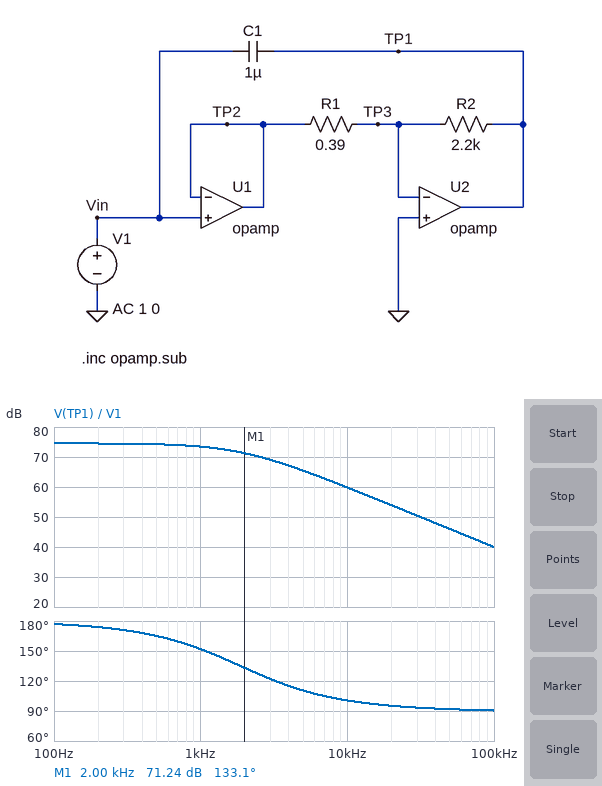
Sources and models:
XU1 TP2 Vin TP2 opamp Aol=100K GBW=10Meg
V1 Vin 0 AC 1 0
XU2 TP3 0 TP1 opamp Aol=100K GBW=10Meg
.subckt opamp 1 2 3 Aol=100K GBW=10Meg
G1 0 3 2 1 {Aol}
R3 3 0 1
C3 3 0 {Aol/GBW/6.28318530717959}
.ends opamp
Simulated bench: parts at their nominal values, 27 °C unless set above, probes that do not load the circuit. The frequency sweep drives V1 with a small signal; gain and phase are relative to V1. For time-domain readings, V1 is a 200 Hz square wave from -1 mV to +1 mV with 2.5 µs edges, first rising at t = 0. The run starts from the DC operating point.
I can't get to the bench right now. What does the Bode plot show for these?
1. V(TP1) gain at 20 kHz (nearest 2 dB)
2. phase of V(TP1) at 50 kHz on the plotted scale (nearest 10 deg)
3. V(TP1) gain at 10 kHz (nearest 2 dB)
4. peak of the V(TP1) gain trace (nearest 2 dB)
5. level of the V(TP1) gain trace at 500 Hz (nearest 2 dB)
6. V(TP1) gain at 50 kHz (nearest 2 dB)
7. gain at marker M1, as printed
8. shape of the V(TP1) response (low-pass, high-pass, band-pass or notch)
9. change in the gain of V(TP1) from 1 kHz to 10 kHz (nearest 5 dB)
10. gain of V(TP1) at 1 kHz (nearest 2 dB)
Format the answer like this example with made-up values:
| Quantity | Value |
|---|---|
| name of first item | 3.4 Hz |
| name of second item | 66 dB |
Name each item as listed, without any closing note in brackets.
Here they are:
| Quantity | Value |
|---|---|
| V(TP1) gain at 20 kHz | 54 dB |
| phase of V(TP1) at 50 kHz on the plotted scale | 90 deg |
| V(TP1) gain at 10 kHz | 60 dB |
| peak of the V(TP1) gain trace | 74 dB |
| level of the V(TP1) gain trace at 500 Hz | 74 dB |
| V(TP1) gain at 50 kHz | 46 dB |
| gain at marker M1, as printed | 71.24 dB |
| shape of the V(TP1) response | low-pass |
| change in the gain of V(TP1) from 1 kHz to 10 kHz | -15 dB |
| gain of V(TP1) at 1 kHz | 74 dB |
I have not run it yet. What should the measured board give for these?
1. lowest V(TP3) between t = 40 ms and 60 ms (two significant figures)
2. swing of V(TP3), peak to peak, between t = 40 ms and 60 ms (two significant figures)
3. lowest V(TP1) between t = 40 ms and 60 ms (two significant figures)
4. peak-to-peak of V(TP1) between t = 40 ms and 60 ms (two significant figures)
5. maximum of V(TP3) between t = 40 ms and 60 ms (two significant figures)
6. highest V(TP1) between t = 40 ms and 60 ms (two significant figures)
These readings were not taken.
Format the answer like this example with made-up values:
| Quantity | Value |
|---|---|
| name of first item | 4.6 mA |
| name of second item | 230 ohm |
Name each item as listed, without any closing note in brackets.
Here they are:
| Quantity | Value |
|---|---|
| lowest V(TP3) between t = 40 ms and 60 ms | -1.9 mV |
| swing of V(TP3), peak to peak, between t = 40 ms and 60 ms | 3.8 mV |
| lowest V(TP1) between t = 40 ms and 60 ms | -5.3 V |
| peak-to-peak of V(TP1) between t = 40 ms and 60 ms | 11 V |
| maximum of V(TP3) between t = 40 ms and 60 ms | 1.9 mV |
| highest V(TP1) between t = 40 ms and 60 ms | 5.3 V |
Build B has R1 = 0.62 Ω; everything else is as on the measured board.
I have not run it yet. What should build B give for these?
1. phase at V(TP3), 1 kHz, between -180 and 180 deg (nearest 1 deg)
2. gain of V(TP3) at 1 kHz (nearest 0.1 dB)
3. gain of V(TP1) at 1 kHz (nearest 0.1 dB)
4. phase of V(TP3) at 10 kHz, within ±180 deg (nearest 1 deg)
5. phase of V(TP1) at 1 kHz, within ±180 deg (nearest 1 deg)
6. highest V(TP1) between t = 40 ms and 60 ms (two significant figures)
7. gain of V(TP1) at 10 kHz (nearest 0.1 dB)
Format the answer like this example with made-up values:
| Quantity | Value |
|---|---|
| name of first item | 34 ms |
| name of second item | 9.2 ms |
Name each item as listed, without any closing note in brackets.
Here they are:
| Quantity | Value |
|---|---|
| phase at V(TP3), 1 kHz, between -180 and 180 deg | 65 deg |
| gain of V(TP3) at 1 kHz | -9.7 dB |
| gain of V(TP1) at 1 kHz | 70.2 dB |
| phase of V(TP3) at 10 kHz, within ±180 deg | 16 deg |
| phase of V(TP1) at 1 kHz, within ±180 deg | 161 deg |
| highest V(TP1) between t = 40 ms and 60 ms | 3.4 V |
| gain of V(TP1) at 10 kHz | 59.6 dB |
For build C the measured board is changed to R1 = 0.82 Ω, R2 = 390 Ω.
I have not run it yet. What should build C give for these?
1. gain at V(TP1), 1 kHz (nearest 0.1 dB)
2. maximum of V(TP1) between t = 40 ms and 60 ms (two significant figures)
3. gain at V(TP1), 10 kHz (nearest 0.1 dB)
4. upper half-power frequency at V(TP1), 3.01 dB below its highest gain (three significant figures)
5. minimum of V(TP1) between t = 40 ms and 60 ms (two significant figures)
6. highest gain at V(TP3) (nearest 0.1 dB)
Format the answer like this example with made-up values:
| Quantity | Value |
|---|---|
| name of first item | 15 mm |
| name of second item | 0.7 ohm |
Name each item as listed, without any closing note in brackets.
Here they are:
| Quantity | Value |
|---|---|
| gain at V(TP1), 1 kHz | 53.5 dB |
| maximum of V(TP1) between t = 40 ms and 60 ms | 470 mV |
| gain at V(TP1), 10 kHz | 52.6 dB |
| upper half-power frequency at V(TP1), 3.01 dB below its highest gain | 21.1 kHz |
| minimum of V(TP1) between t = 40 ms and 60 ms | -470 mV |
| highest gain at V(TP3) | 0 dB |
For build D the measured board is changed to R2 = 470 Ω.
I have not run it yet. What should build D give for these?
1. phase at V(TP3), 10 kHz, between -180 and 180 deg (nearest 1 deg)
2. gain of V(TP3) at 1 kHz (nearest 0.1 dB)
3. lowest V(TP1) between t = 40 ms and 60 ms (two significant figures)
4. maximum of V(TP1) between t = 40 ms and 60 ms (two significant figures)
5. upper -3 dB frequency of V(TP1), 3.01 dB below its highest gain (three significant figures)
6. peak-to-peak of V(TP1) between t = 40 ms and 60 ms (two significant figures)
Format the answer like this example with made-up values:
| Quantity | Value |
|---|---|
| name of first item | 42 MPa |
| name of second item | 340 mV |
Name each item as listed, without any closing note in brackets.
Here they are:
| Quantity | Value |
|---|---|
| phase at V(TP3), 10 kHz, between -180 and 180 deg | 39 deg |
| gain of V(TP3) at 1 kHz | -18.5 dB |
| lowest V(TP1) between t = 40 ms and 60 ms | -1.2 V |
| maximum of V(TP1) between t = 40 ms and 60 ms | 1.2 V |
| upper -3 dB frequency of V(TP1), 3.01 dB below its highest gain | 8.39 kHz |
| peak-to-peak of V(TP1) between t = 40 ms and 60 ms | 2.4 V |
